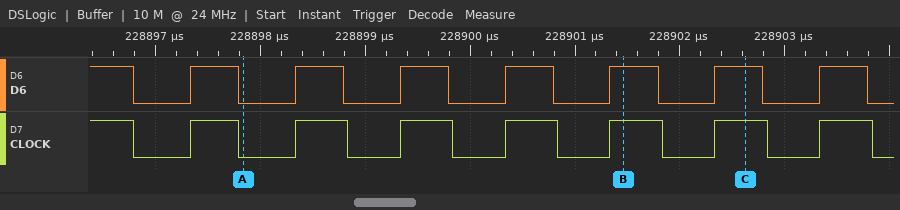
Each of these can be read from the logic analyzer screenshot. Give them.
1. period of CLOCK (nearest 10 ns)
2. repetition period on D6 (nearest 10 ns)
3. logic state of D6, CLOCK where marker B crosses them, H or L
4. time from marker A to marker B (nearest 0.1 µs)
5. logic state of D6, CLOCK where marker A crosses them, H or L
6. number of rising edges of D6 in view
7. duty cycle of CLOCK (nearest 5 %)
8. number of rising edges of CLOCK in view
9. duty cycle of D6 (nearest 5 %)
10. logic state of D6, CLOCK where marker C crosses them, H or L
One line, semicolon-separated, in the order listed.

1000 ns; 1000 ns; D6=H, CLOCK=H; 3.6 µs; D6=L, CLOCK=L; 7; 50 %; 7; 45 %; D6=H, CLOCK=H
